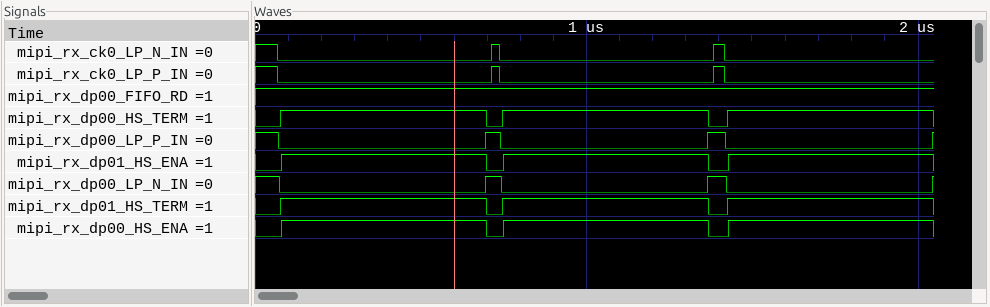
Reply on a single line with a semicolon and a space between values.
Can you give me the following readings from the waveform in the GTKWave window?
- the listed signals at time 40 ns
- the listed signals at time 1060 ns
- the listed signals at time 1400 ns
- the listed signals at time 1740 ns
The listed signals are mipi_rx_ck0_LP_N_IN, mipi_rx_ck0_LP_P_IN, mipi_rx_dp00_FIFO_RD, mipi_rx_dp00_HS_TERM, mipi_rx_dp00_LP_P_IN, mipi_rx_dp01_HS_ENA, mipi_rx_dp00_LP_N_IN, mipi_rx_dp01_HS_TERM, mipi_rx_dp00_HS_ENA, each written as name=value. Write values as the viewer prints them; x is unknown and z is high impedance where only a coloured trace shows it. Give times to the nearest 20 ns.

mipi_rx_ck0_LP_N_IN=1, mipi_rx_ck0_LP_P_IN=1, mipi_rx_dp00_FIFO_RD=1, mipi_rx_dp00_HS_TERM=0, mipi_rx_dp00_LP_P_IN=1, mipi_rx_dp01_HS_ENA=0, mipi_rx_dp00_LP_N_IN=1, mipi_rx_dp01_HS_TERM=0, mipi_rx_dp00_HS_ENA=0; mipi_rx_ck0_LP_N_IN=0, mipi_rx_ck0_LP_P_IN=0, mipi_rx_dp00_FIFO_RD=1, mipi_rx_dp00_HS_TERM=1, mipi_rx_dp00_LP_P_IN=0, mipi_rx_dp01_HS_ENA=1, mipi_rx_dp00_LP_N_IN=0, mipi_rx_dp01_HS_TERM=1, mipi_rx_dp00_HS_ENA=1; mipi_rx_ck0_LP_N_IN=1, mipi_rx_ck0_LP_P_IN=1, mipi_rx_dp00_FIFO_RD=1, mipi_rx_dp00_HS_TERM=0, mipi_rx_dp00_LP_P_IN=1, mipi_rx_dp01_HS_ENA=0, mipi_rx_dp00_LP_N_IN=1, mipi_rx_dp01_HS_TERM=0, mipi_rx_dp00_HS_ENA=0; mipi_rx_ck0_LP_N_IN=0, mipi_rx_ck0_LP_P_IN=0, mipi_rx_dp00_FIFO_RD=1, mipi_rx_dp00_HS_TERM=1, mipi_rx_dp00_LP_P_IN=0, mipi_rx_dp01_HS_ENA=1, mipi_rx_dp00_LP_N_IN=0, mipi_rx_dp01_HS_TERM=1, mipi_rx_dp00_HS_ENA=1
